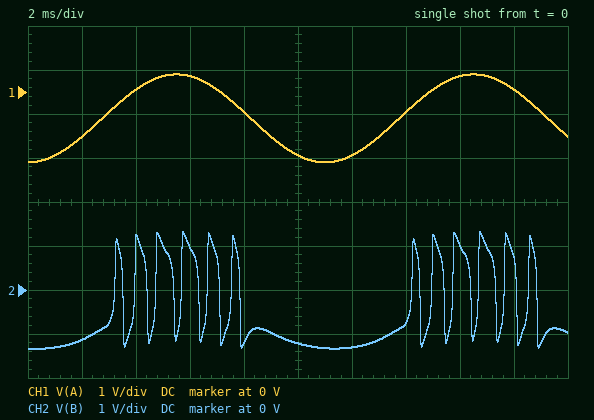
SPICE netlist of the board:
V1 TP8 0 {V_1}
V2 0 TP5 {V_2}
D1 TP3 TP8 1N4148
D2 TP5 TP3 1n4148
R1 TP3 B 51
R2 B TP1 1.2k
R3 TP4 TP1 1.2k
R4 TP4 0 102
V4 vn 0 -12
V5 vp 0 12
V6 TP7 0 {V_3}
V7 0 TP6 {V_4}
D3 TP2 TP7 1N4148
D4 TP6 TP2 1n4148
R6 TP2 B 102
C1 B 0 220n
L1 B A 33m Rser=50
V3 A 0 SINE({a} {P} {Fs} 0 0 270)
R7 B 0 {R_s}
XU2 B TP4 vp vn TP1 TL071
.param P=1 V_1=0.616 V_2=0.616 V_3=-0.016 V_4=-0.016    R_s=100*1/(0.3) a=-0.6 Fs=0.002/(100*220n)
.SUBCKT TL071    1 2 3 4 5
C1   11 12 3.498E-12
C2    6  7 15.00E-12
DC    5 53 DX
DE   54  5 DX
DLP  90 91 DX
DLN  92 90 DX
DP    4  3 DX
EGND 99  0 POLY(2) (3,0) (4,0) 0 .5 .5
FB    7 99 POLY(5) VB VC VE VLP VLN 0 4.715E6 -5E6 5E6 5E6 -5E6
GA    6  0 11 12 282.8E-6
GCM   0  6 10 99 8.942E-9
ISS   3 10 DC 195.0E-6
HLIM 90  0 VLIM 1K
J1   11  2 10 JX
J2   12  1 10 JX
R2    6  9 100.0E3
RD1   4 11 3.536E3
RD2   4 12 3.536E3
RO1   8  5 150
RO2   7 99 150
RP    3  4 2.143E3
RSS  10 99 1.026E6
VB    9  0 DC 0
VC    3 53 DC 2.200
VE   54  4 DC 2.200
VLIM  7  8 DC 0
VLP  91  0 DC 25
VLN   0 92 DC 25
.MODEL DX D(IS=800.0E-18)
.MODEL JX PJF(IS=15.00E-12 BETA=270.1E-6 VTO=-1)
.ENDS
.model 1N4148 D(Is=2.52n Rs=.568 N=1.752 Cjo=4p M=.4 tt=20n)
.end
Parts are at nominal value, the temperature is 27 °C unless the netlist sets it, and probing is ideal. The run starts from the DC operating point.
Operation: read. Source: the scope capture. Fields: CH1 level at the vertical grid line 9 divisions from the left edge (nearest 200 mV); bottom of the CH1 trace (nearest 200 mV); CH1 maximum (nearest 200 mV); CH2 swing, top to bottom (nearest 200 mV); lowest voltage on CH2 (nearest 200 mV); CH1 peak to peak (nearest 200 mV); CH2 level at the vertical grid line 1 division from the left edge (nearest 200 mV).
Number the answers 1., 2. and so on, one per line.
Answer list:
1. 0 V
2. -1.6 V
3. 400 mV
4. 2.6 V
5. -1.4 V
6. 2.0 V
7. -1.2 V
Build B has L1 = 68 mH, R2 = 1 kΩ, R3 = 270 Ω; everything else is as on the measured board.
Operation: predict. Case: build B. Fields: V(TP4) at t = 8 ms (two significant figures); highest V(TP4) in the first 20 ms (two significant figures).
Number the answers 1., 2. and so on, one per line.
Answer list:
1. -420 mV
2. 390 mV
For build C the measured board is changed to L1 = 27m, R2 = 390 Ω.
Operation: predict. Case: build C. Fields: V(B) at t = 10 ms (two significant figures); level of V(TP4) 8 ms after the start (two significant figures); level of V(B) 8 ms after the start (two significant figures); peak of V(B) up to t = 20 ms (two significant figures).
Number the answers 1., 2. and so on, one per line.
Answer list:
1. -1.5 V
2. -700 mV
3. -1.6 V
4. 2.0 V
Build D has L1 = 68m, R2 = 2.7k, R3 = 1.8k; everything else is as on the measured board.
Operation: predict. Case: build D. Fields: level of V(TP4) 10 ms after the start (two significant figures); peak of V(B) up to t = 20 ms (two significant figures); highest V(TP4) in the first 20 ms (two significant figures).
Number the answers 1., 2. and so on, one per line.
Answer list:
1. -560 mV
2. 920 mV
3. 560 mV
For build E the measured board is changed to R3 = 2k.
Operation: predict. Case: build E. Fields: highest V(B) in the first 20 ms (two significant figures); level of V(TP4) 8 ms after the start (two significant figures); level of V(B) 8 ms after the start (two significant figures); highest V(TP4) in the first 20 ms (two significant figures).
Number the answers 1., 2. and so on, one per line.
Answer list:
1. 1.3 V
2. -510 mV
3. -630 mV
4. 510 mV
